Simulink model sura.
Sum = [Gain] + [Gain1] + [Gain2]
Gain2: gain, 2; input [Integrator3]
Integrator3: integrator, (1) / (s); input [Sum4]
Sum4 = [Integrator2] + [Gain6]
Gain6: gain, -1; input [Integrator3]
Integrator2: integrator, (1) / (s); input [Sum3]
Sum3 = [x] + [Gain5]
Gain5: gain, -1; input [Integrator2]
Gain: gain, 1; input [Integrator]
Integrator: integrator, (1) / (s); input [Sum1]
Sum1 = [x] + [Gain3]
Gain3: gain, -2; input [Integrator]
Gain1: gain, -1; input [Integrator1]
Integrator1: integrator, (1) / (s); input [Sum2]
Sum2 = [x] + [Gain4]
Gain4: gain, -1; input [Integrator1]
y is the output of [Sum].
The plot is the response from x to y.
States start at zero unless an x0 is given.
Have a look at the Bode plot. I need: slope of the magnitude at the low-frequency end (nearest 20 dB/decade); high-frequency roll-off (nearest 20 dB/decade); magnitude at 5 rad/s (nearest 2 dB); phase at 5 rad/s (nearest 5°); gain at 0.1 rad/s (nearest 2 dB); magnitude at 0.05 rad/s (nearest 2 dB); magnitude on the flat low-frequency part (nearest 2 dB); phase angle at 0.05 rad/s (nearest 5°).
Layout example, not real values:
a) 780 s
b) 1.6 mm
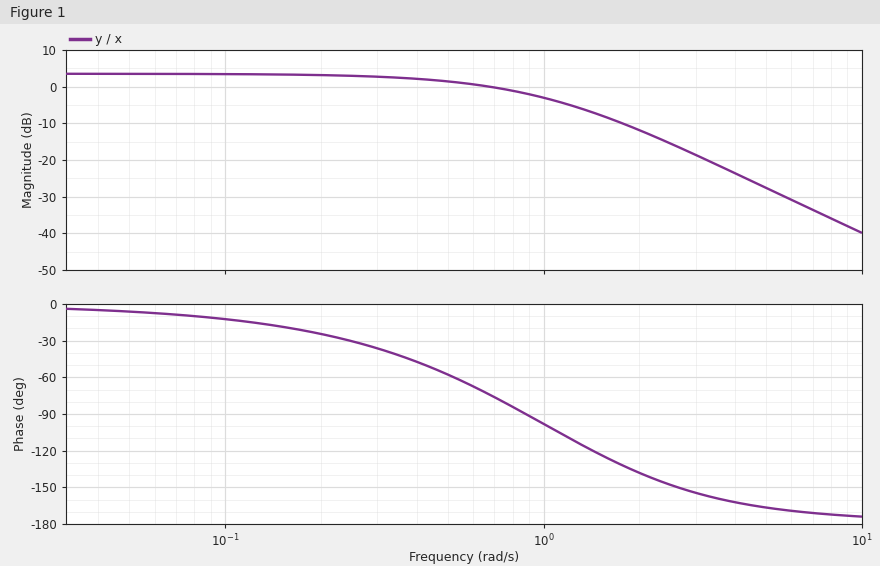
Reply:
a) 0 dB/decade
b) -40 dB/decade
c) -28 dB
d) -165°
e) 4 dB
f) 4 dB
g) 4 dB
h) -5°
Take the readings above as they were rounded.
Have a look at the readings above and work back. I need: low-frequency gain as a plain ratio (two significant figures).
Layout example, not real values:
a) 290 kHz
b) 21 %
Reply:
a) 1.6
